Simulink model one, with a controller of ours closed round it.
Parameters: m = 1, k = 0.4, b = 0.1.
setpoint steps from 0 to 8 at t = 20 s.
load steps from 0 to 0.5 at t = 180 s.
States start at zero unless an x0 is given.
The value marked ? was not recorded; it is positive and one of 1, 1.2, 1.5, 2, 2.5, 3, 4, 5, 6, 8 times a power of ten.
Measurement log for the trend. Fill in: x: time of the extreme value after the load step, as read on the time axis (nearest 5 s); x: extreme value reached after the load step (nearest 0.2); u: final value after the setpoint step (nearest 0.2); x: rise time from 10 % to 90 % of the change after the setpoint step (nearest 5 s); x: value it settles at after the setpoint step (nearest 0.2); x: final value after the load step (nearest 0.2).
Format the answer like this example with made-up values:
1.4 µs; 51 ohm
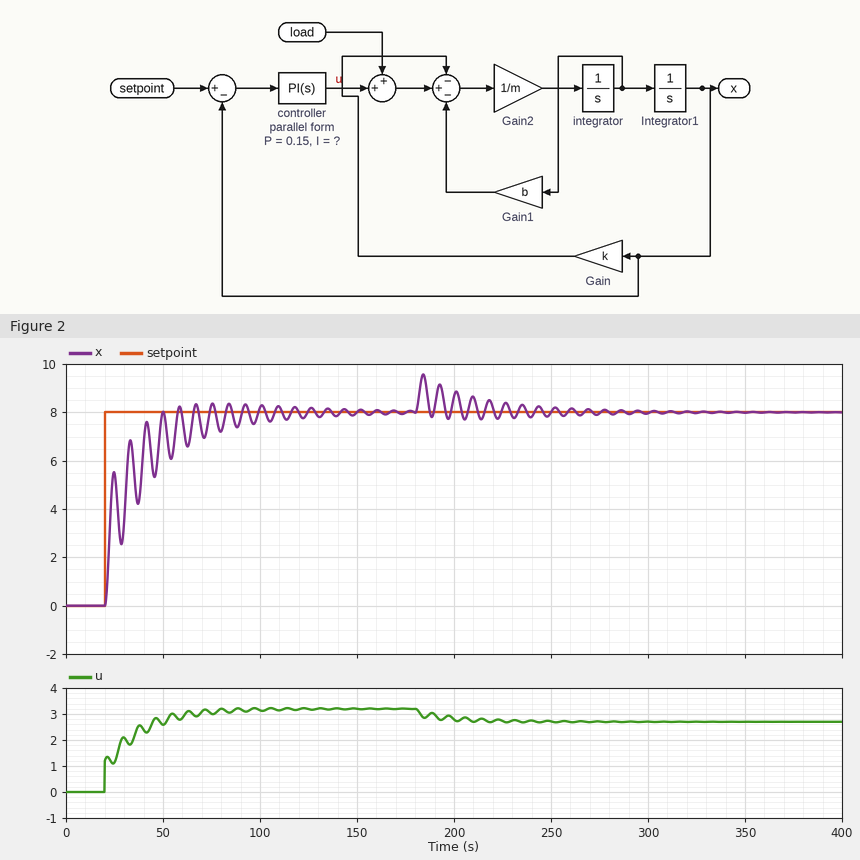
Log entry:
185 s; 9.6; 3.2; 20 s; 8.0; 8.0
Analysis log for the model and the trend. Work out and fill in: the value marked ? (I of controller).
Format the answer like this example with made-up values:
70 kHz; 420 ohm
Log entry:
0.03
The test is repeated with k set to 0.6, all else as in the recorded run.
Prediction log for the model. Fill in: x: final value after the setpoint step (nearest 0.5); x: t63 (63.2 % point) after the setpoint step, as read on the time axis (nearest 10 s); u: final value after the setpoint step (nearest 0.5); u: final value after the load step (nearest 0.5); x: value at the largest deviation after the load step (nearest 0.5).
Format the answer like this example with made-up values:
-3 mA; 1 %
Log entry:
8.0; 30 s; 5.0; 4.5; 9.0
